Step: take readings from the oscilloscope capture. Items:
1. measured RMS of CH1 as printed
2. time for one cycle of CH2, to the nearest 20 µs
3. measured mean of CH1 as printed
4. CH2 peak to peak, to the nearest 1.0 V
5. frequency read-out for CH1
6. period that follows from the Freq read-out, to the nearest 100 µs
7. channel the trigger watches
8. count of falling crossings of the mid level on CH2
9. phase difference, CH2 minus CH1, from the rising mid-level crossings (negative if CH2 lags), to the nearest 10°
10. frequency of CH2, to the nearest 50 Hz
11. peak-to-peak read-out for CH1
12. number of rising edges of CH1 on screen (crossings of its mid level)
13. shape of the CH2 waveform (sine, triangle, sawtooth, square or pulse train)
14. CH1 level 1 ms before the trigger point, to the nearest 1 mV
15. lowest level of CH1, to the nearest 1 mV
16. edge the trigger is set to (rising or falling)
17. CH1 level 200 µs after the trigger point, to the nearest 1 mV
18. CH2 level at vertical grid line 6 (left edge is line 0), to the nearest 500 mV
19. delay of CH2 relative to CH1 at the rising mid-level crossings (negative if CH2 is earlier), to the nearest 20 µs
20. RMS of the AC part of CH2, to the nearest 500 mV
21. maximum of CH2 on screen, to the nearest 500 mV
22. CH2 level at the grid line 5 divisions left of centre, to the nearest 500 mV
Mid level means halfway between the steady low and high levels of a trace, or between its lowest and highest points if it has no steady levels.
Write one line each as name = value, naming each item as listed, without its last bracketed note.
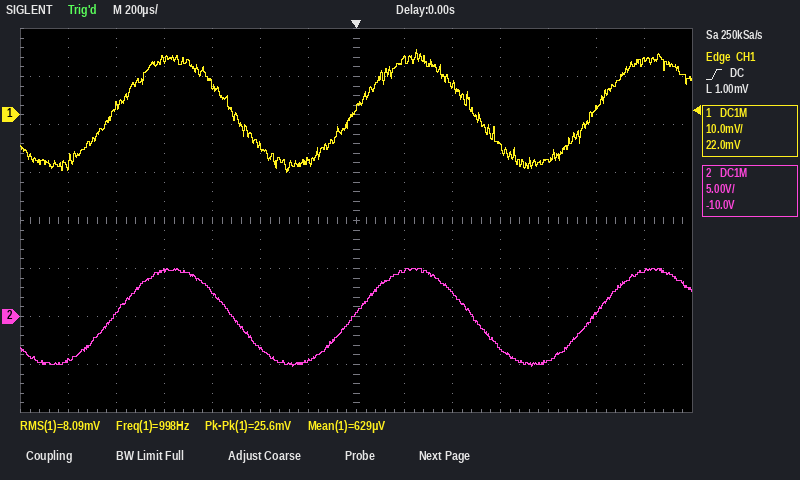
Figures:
measured RMS of CH1 as printed = 8.09 mV
time for one cycle of CH2, to the nearest 20 µs = 1.00 ms
measured mean of CH1 as printed = 629 µV
CH2 peak to peak, to the nearest 1.0 V = 10.0 V
frequency read-out for CH1 = 998 Hz
period that follows from the Freq read-out, to the nearest 100 µs = 1.0 ms
channel the trigger watches = CH1
count of falling crossings of the mid level on CH2 = 2
phase difference, CH2 minus CH1, from the rising mid-level crossings (negative if CH2 lags), to the nearest 10° = 0°
frequency of CH2, to the nearest 50 Hz = 1.00 kHz
peak-to-peak read-out for CH1 = 25.6 mV
number of rising edges of CH1 on screen = 3
shape of the CH2 waveform = sine
CH1 level 1 ms before the trigger point, to the nearest 1 mV = 2 mV
lowest level of CH1, to the nearest 1 mV = -12 mV
edge the trigger is set to = rising
CH1 level 200 µs after the trigger point, to the nearest 1 mV = 12 mV
CH2 level at vertical grid line 6 (left edge is line 0), to the nearest 500 mV = -4.5 V
delay of CH2 relative to CH1 at the rising mid-level crossings (negative if CH2 is earlier), to the nearest 20 µs = 0 µs
RMS of the AC part of CH2, to the nearest 500 mV = 3.5 V
maximum of CH2 on screen, to the nearest 500 mV = 5.0 V
CH2 level at the grid line 5 divisions left of centre, to the nearest 500 mV = 500 mV
